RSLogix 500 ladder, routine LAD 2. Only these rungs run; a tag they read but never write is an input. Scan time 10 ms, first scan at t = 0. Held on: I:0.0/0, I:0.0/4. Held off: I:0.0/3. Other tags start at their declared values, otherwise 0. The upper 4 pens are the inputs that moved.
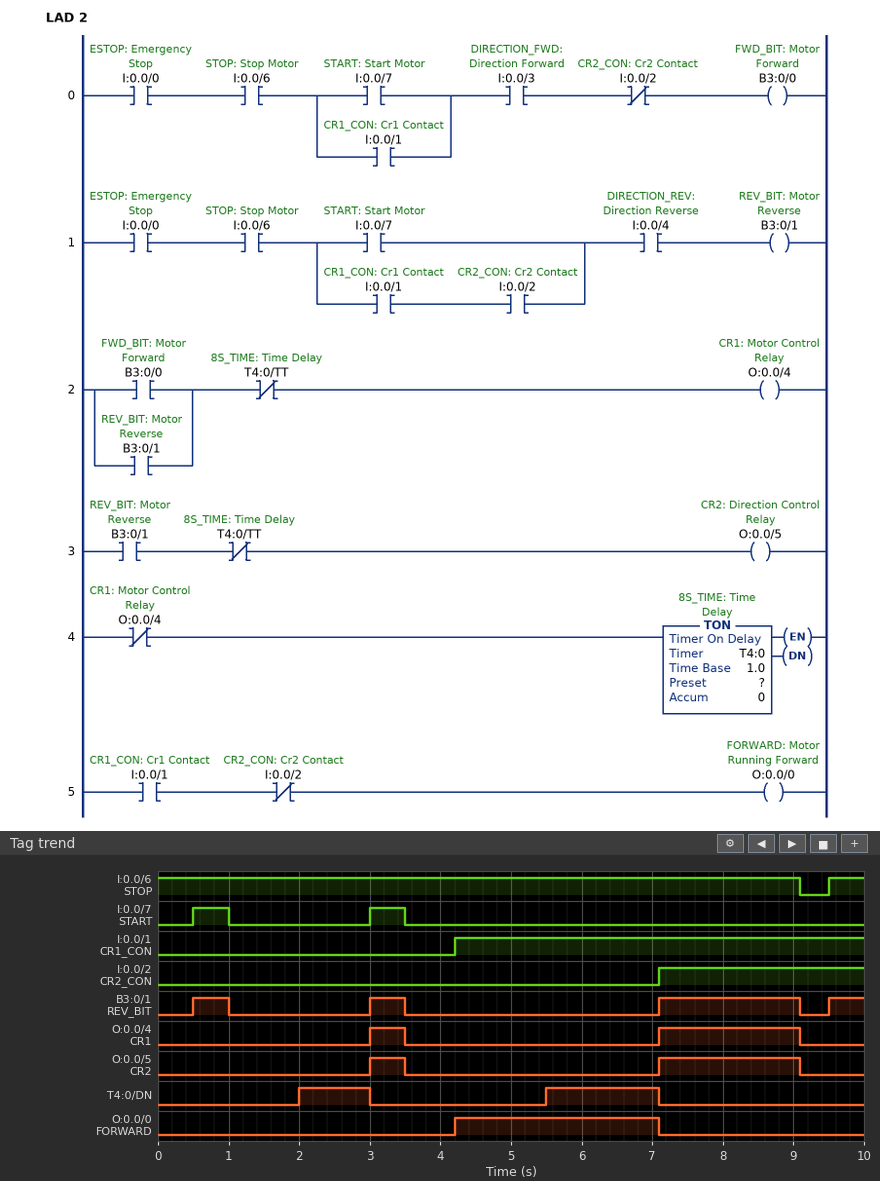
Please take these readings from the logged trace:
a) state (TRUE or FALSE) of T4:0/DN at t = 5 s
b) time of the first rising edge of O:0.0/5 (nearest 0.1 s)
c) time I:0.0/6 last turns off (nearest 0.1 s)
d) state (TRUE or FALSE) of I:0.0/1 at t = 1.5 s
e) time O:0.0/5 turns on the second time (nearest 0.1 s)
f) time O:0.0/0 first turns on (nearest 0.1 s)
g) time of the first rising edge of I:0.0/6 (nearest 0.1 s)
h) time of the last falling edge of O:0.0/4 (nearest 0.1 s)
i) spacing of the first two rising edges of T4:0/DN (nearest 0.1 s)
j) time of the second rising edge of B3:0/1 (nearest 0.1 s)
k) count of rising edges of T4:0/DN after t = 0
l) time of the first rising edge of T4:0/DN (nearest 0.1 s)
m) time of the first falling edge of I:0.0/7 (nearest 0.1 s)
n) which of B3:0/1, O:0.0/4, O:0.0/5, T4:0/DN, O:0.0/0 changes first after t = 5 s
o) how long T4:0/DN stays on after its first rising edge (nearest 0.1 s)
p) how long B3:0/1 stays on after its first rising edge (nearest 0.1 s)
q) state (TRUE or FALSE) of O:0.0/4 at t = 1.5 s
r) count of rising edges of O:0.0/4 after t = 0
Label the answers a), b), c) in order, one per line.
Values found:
a) FALSE
b) 3.0 s
c) 9.1 s
d) FALSE
e) 7.1 s
f) 4.2 s
g) 9.5 s
h) 9.1 s
i) 3.5 s
j) 3.0 s
k) 2
l) 2.0 s
m) 1.0 s
n) T4:0/DN
o) 1.0 s
p) 0.5 s
q) FALSE
r) 2
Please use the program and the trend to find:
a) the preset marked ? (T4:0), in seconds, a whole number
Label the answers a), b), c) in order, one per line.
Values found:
a) 2 s
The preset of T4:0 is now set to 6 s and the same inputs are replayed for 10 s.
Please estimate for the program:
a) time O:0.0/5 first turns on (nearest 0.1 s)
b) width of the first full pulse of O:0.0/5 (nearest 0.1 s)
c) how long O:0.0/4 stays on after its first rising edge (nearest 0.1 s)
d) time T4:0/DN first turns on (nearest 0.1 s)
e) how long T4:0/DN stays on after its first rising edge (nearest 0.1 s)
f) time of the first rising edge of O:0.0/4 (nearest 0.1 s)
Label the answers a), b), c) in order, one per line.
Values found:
a) 7.1 s
b) 2.0 s
c) 2.0 s
d) 6.0 s
e) 1.1 s
f) 7.1 s
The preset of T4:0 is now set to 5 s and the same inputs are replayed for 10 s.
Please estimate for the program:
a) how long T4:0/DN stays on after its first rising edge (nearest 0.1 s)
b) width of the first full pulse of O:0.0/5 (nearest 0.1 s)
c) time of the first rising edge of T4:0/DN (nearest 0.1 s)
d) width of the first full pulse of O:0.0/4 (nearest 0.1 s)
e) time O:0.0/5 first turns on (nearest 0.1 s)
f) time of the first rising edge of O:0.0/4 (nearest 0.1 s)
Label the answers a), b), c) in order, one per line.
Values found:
a) 2.1 s
b) 2.0 s
c) 5.0 s
d) 2.0 s
e) 7.1 s
f) 7.1 s
